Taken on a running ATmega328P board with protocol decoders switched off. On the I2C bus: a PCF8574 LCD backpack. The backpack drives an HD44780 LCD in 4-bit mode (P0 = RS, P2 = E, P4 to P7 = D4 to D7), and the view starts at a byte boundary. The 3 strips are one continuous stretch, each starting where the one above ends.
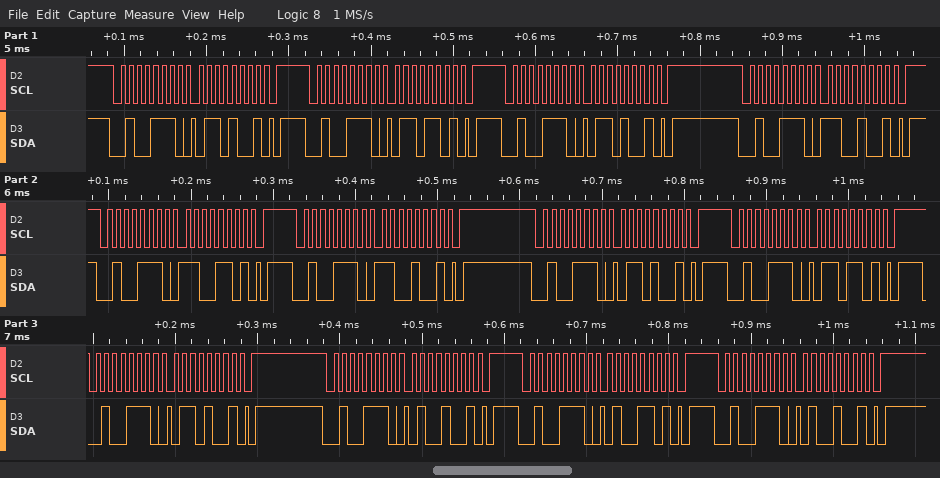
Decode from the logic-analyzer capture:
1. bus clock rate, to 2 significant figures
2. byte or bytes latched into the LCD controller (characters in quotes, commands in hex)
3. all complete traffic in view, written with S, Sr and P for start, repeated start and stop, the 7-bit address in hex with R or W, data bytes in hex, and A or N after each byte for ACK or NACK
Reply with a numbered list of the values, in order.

1. 100 kHz
2. 'l' 'd'
3. S 27W A 69 A P S 27W A 6D A P S 27W A 69 A P S 27W A C9 A P S 27W A CD A P S 27W A C9 A P S 27W A 69 A P S 27W A 6D A P S 27W A 69 A P S 27W A 49 A P S 27W A 4D A P S 27W A 49 A P
